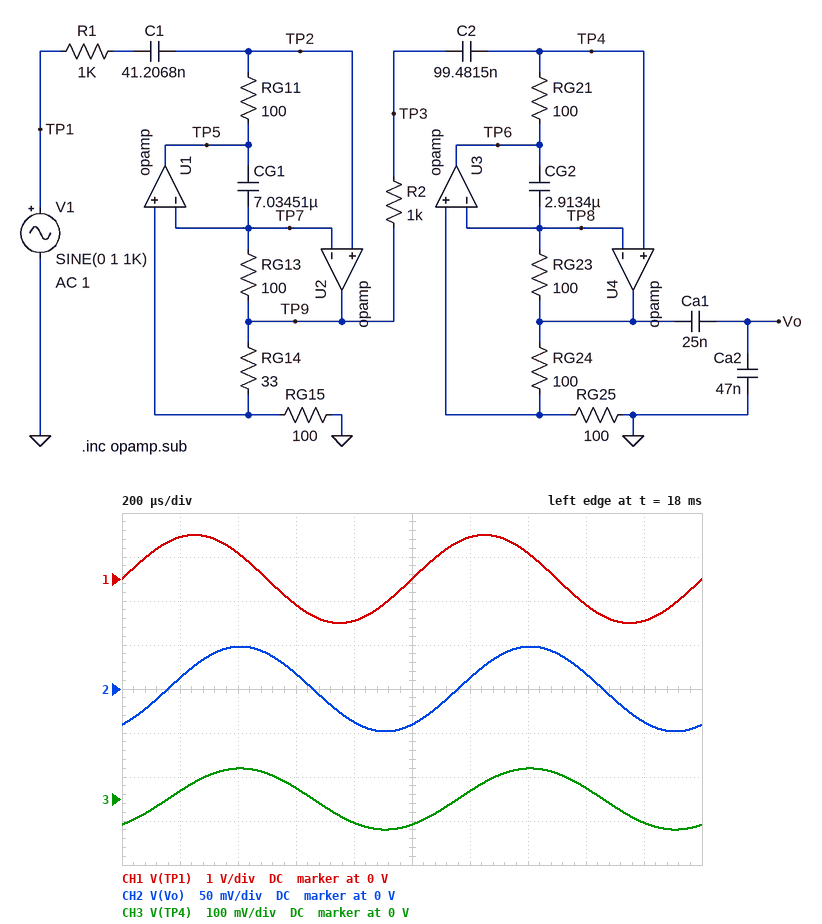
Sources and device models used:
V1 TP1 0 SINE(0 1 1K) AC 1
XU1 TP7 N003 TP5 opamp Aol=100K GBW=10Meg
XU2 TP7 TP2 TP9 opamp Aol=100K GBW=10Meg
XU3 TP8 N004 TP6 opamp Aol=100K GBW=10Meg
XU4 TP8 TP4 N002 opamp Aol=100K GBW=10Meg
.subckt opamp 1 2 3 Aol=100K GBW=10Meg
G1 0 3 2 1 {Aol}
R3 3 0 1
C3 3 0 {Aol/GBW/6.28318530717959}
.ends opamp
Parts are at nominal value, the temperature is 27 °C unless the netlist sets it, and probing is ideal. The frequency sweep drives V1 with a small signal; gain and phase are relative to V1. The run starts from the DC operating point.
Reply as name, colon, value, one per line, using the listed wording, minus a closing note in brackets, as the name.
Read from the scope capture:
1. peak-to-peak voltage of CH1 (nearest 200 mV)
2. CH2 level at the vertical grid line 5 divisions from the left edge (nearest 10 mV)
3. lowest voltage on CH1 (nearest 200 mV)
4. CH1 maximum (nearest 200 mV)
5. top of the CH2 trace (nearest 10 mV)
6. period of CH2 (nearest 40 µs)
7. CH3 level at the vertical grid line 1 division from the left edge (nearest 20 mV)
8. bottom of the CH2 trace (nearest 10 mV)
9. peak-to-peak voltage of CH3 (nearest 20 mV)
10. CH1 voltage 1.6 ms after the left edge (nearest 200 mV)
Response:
peak-to-peak voltage of CH1: 2.0 V
CH2 level at the vertical grid line 5 divisions from the left edge: -40 mV
lowest voltage on CH1: -1.0 V
CH1 maximum: 1.0 V
top of the CH2 trace: 50 mV
period of CH2: 1.00 ms
CH3 level at the vertical grid line 1 division from the left edge: 20 mV
bottom of the CH2 trace: -50 mV
peak-to-peak voltage of CH3: 140 mV
CH1 voltage 1.6 ms after the left edge: -600 mV
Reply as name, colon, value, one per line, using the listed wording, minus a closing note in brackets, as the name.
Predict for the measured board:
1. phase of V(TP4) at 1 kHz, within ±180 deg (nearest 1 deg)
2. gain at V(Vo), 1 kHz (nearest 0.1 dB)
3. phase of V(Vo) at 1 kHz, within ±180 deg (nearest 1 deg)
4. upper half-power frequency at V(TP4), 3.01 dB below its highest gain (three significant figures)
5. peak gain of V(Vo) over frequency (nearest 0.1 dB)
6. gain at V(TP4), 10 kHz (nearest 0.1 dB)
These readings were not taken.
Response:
phase of V(TP4) at 1 kHz, within ±180 deg: -57 deg
gain at V(Vo), 1 kHz: -26.3 dB
phase of V(Vo) at 1 kHz, within ±180 deg: -57 deg
upper half-power frequency at V(TP4), 3.01 dB below its highest gain: 372 kHz
peak gain of V(Vo) over frequency: -0.7 dB
gain at V(TP4), 10 kHz: 2.2 dB
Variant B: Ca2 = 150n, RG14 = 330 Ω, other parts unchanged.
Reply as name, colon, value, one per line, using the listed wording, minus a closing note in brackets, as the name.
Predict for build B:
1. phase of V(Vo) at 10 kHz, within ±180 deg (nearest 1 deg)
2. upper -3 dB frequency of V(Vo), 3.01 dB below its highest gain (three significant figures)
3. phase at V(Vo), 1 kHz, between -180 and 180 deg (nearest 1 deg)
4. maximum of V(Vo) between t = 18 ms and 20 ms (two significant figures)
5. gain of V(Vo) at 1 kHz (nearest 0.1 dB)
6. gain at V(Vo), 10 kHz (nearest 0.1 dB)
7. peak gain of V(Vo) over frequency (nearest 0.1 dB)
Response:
phase of V(Vo) at 10 kHz, within ±180 deg: 74 deg
upper -3 dB frequency of V(Vo), 3.01 dB below its highest gain: 188 kHz
phase at V(Vo), 1 kHz, between -180 and 180 deg: -50 deg
maximum of V(Vo) between t = 18 ms and 20 ms: 4.5 mV
gain of V(Vo) at 1 kHz: -46.9 dB
gain at V(Vo), 10 kHz: 1.2 dB
peak gain of V(Vo) over frequency: 1.9 dB
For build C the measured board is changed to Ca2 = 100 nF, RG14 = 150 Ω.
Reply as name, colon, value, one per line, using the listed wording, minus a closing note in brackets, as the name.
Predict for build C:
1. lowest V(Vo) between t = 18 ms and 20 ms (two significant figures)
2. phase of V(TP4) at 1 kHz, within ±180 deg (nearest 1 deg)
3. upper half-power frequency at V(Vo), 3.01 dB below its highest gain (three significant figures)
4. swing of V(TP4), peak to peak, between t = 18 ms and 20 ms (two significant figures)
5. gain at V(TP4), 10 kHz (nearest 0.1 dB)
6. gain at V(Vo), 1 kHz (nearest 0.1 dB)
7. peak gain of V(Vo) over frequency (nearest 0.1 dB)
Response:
lowest V(Vo) between t = 18 ms and 20 ms: -8.4 mV
phase of V(TP4) at 1 kHz, within ±180 deg: -51 deg
upper half-power frequency at V(Vo), 3.01 dB below its highest gain: 266 kHz
swing of V(TP4), peak to peak, between t = 18 ms and 20 ms: 42 mV
gain at V(TP4), 10 kHz: 8.1 dB
gain at V(Vo), 1 kHz: -41.5 dB
peak gain of V(Vo) over frequency: 0.1 dB
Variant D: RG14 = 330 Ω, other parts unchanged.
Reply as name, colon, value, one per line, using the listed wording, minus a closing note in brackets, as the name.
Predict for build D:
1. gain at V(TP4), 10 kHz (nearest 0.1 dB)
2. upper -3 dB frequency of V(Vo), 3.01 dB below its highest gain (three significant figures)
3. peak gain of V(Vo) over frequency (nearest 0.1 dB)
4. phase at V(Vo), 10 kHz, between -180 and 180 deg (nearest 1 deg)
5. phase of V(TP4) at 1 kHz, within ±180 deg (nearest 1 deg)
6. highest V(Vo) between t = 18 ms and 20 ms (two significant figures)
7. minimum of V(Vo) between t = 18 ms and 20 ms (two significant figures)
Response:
gain at V(TP4), 10 kHz: 12.1 dB
upper -3 dB frequency of V(Vo), 3.01 dB below its highest gain: 188 kHz
peak gain of V(Vo) over frequency: 9.6 dB
phase at V(Vo), 10 kHz, between -180 and 180 deg: 74 deg
phase of V(TP4) at 1 kHz, within ±180 deg: -50 deg
highest V(Vo) between t = 18 ms and 20 ms: 11 mV
minimum of V(Vo) between t = 18 ms and 20 ms: -11 mV
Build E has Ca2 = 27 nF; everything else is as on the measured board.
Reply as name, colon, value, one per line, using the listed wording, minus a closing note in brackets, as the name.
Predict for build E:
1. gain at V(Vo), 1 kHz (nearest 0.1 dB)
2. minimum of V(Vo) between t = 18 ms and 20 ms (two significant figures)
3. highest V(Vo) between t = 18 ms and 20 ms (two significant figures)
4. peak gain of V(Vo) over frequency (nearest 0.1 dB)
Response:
gain at V(Vo), 1 kHz: -23.5 dB
minimum of V(Vo) between t = 18 ms and 20 ms: -67 mV
highest V(Vo) between t = 18 ms and 20 ms: 67 mV
peak gain of V(Vo) over frequency: 2.1 dB
